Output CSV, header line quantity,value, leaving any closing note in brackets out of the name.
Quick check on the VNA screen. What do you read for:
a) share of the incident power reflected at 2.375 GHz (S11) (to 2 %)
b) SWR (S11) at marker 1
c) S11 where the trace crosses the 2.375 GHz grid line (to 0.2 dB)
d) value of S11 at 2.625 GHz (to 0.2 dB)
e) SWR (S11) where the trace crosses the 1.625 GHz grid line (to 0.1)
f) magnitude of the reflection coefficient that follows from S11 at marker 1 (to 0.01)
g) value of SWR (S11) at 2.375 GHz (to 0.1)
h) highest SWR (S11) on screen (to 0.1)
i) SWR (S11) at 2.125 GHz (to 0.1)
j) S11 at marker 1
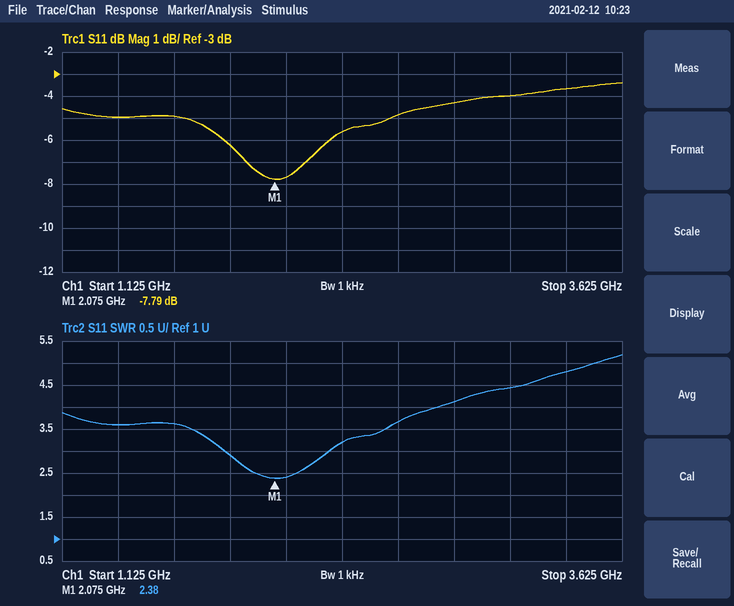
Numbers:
quantity,value
share of the incident power reflected at 2.375 GHz (S11),28 %
SWR (S11) at marker 1,2.38
S11 where the trace crosses the 2.375 GHz grid line,-5.6 dB
value of S11 at 2.625 GHz,-4.8 dB
SWR (S11) where the trace crosses the 1.625 GHz grid line,3.6
magnitude of the reflection coefficient that follows from S11 at marker 1,0.41
value of SWR (S11) at 2.375 GHz,3.2
highest SWR (S11) on screen,5.2
SWR (S11) at 2.125 GHz,2.4
S11 at marker 1,-7.79 dB
